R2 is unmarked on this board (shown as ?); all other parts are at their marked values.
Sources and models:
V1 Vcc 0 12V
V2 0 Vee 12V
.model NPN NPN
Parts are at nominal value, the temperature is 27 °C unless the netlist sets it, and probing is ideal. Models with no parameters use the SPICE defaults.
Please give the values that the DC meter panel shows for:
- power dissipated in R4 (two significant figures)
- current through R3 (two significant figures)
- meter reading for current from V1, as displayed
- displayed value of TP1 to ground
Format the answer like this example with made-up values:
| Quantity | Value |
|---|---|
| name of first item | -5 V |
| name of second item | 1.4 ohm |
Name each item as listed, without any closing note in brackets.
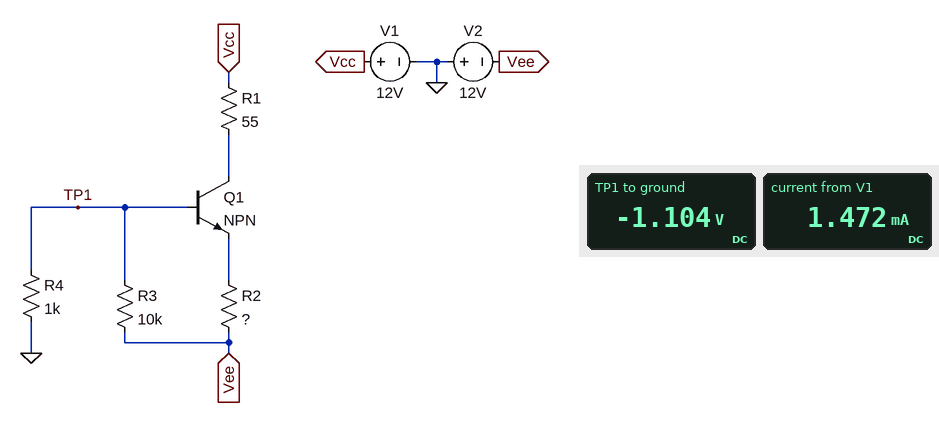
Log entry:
| Quantity | Value |
|---|---|
| power dissipated in R4 | 1.2 mW |
| current through R3 | 1.1 mA |
| meter reading for current from V1, as displayed | 1.472 mA |
| displayed value of TP1 to ground | -1.104 V |
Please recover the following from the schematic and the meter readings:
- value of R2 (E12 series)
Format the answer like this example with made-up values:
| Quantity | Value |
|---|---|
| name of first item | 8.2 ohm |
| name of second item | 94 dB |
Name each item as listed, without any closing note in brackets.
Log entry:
| Quantity | Value |
|---|---|
| value of R2 | 6.8 kΩ |
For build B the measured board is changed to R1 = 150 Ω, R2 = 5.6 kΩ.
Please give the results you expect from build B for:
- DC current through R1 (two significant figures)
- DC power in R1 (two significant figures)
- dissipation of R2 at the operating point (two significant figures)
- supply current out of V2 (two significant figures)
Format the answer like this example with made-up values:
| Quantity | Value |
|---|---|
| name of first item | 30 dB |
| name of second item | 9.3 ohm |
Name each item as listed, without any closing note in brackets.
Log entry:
| Quantity | Value |
|---|---|
| DC current through R1 | 1.8 mA |
| DC power in R1 | 480 µW |
| dissipation of R2 at the operating point | 18 mW |
| supply current out of V2 | 2.9 mA |
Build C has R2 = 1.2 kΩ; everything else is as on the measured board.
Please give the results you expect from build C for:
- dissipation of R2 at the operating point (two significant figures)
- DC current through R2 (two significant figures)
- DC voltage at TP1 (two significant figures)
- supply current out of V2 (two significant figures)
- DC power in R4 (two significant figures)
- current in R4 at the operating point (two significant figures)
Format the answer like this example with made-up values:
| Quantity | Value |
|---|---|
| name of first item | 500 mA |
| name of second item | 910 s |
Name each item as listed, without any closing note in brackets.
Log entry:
| Quantity | Value |
|---|---|
| dissipation of R2 at the operating point | 83 mW |
| DC current through R2 | 8.3 mA |
| DC voltage at TP1 | -1.2 V |
| supply current out of V2 | 9.4 mA |
| DC power in R4 | 1.4 mW |
| current in R4 at the operating point | 1.2 mA |
